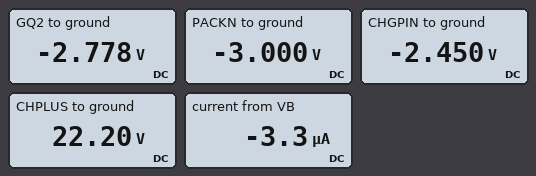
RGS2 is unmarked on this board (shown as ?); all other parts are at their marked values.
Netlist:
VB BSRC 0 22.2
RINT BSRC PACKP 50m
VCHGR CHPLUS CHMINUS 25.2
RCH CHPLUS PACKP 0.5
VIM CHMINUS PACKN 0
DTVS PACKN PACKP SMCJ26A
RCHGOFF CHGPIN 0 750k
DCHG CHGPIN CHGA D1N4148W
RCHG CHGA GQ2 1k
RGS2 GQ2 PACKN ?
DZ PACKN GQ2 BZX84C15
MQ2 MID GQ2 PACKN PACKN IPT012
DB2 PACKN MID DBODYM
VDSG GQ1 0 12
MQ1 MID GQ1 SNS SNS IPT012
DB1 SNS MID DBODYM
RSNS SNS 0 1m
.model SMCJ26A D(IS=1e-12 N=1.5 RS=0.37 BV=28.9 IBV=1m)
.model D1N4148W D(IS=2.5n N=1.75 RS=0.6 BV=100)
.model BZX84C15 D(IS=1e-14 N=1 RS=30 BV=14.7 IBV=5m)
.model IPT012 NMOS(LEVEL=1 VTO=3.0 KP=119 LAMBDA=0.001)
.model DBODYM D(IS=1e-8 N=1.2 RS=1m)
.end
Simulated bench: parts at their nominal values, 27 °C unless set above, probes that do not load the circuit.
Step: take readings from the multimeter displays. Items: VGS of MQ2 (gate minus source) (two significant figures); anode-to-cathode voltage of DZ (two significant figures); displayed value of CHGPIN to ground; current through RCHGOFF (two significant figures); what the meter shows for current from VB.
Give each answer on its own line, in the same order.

220 mV
-220 mV
-2.450 V
3.3 µA
-3.3 µA
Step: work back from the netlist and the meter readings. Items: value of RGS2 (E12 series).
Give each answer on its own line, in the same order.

68 kΩ
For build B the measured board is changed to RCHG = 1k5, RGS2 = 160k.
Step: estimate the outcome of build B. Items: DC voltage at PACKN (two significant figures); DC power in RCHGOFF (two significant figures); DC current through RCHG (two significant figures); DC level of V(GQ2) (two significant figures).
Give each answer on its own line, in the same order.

-3.0 V
6.5 µW
2.9 µA
-2.5 V
